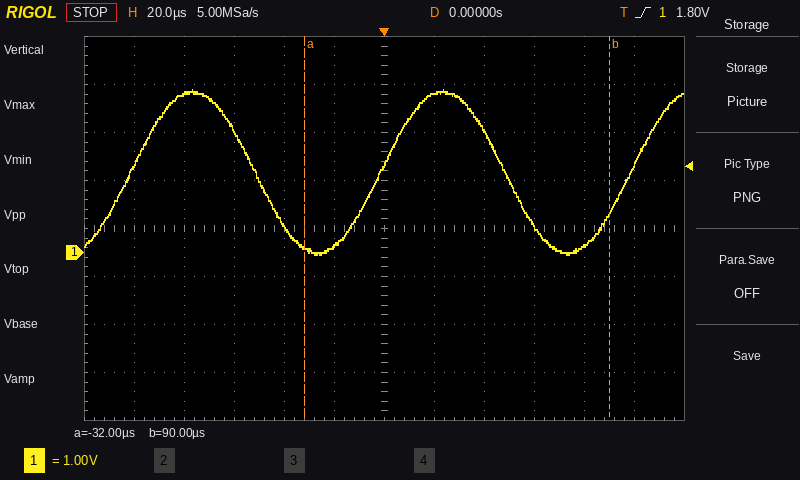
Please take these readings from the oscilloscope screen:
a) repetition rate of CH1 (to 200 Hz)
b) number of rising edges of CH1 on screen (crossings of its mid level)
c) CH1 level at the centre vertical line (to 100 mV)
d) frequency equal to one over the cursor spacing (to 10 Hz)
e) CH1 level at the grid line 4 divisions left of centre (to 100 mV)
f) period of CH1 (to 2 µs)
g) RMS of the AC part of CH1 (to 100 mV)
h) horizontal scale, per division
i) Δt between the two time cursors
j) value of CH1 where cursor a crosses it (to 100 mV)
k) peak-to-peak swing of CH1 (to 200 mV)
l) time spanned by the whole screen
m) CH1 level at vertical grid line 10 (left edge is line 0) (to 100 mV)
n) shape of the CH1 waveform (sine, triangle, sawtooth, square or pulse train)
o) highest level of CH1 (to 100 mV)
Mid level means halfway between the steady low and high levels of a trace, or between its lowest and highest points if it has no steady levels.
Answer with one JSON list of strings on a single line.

["10.0 kHz", "3", "1.8 V", "8.20 kHz", "3.3 V", "100 µs", "1.2 V", "20 µs", "122 µs", "100 mV", "3.4 V", "240 µs", "100 mV", "sine", "3.4 V"]
